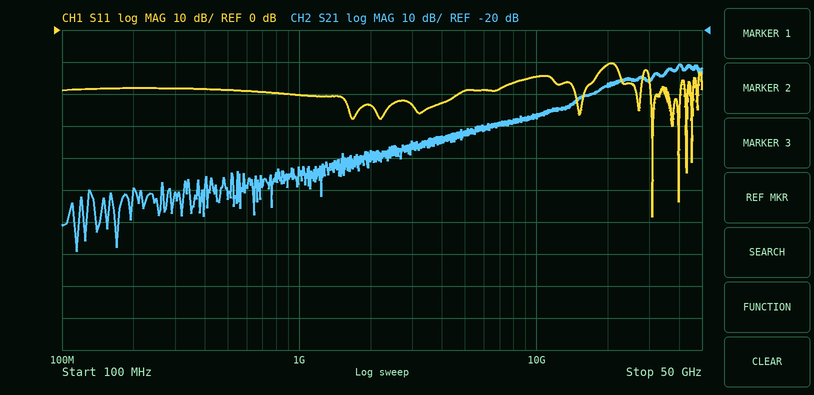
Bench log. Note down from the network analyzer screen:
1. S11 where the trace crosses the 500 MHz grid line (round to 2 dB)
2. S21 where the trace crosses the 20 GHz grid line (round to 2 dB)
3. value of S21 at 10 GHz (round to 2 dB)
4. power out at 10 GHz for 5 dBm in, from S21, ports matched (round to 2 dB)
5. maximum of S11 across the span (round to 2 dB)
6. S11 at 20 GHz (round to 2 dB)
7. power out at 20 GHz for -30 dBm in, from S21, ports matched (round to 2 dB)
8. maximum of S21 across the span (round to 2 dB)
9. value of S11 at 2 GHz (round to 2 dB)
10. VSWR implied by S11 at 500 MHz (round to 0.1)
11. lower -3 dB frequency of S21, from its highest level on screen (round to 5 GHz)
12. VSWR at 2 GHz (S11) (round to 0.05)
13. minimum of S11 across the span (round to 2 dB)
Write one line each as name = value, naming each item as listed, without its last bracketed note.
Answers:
S11 where the trace crosses the 500 MHz grid line = -18 dB
S21 where the trace crosses the 20 GHz grid line = -38 dB
value of S21 at 10 GHz = -46 dB
power out at 10 GHz for 5 dBm in, from S21, ports matched = -42 dBm
maximum of S11 across the span = -10 dB
S11 at 20 GHz = -10 dB
power out at 20 GHz for -30 dBm in, from S21, ports matched = -68 dBm
maximum of S21 across the span = -30 dB
value of S11 at 2 GHz = -24 dB
VSWR implied by S11 at 500 MHz = 1.3
lower -3 dB frequency of S21, from its highest level on screen = 35 GHz
VSWR at 2 GHz (S11) = 1.15
minimum of S11 across the span = -58 dB
